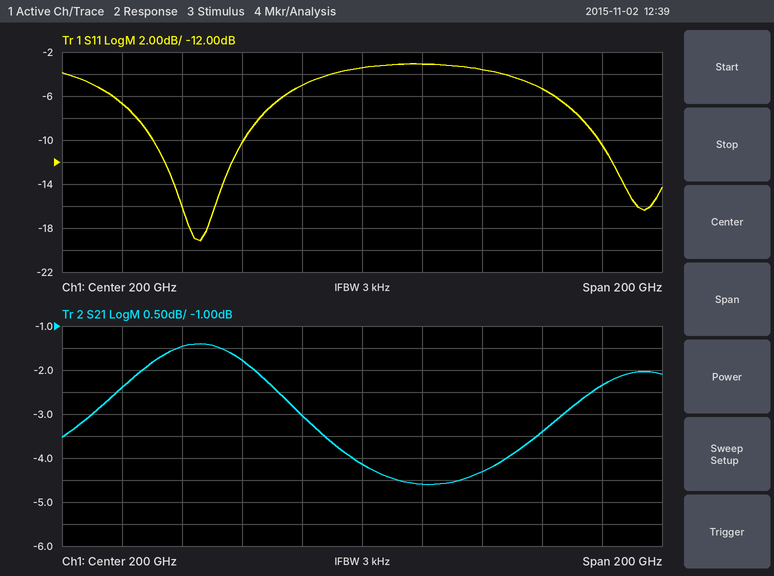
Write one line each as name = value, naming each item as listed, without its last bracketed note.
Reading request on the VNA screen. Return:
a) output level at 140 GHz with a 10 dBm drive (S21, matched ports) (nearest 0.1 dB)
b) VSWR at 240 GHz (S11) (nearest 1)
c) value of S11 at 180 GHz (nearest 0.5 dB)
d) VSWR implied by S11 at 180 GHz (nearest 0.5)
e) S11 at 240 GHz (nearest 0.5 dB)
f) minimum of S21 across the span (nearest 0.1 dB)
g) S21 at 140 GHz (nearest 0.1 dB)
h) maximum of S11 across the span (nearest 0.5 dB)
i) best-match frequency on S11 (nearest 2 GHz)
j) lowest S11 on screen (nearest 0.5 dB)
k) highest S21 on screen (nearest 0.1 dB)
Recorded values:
output level at 140 GHz with a 10 dBm drive (S21, matched ports) = 8.5 dBm
VSWR at 240 GHz (S11) = 5
value of S11 at 180 GHz = -5.0 dB
VSWR implied by S11 at 180 GHz = 3.5
S11 at 240 GHz = -3.5 dB
minimum of S21 across the span = -4.6 dB
S21 at 140 GHz = -1.5 dB
maximum of S11 across the span = -3.0 dB
best-match frequency on S11 = 146 GHz
lowest S11 on screen = -19.0 dB
highest S21 on screen = -1.4 dB
